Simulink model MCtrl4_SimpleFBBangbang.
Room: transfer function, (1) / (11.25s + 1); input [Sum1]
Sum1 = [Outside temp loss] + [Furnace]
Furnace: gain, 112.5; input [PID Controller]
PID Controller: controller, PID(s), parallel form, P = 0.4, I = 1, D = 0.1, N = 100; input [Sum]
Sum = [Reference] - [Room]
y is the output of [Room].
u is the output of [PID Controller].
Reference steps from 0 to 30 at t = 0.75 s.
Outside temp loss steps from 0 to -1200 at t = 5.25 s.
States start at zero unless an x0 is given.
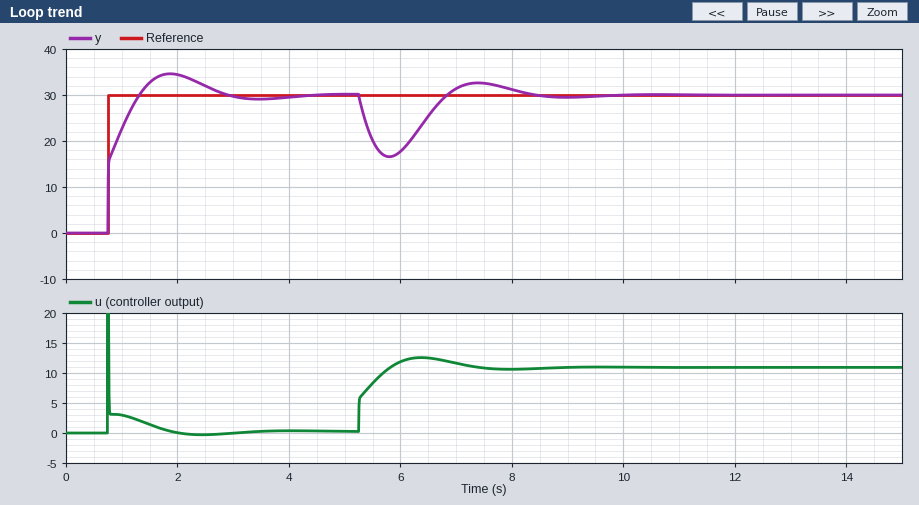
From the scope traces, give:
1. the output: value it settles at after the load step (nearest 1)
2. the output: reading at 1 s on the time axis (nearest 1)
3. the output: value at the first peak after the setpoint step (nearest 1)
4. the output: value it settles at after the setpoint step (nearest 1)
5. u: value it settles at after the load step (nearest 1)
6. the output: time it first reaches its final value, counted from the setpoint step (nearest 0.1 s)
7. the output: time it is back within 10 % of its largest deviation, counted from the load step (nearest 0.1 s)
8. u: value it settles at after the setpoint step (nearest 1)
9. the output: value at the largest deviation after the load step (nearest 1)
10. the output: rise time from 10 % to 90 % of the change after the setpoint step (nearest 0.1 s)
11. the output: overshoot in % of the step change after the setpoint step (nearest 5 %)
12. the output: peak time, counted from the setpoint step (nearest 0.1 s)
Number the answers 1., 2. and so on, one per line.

1. 30
2. 23
3. 35
4. 30
5. 11
6. 0.6 s
7. 2.7 s
8. 0
9. 17
10. 0.4 s
11. 15 %
12. 1.1 s
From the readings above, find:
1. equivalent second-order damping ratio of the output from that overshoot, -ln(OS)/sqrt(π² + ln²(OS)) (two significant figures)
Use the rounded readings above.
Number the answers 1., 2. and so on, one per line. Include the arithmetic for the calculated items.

1. ln(0.15) = -1.897; 1.897 / sqrt(9.870 + 3.599) = 0.52
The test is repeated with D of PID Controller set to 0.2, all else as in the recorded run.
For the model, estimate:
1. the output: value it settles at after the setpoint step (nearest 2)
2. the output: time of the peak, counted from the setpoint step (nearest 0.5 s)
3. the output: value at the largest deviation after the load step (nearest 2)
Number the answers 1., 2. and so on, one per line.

1. 30
2. 1.5 s
3. 18
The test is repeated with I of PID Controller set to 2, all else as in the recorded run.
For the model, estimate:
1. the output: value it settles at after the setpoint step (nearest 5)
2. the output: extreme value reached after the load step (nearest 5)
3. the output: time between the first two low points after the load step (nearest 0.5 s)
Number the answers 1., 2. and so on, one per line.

1. 30
2. 20
3. 2.0 s
